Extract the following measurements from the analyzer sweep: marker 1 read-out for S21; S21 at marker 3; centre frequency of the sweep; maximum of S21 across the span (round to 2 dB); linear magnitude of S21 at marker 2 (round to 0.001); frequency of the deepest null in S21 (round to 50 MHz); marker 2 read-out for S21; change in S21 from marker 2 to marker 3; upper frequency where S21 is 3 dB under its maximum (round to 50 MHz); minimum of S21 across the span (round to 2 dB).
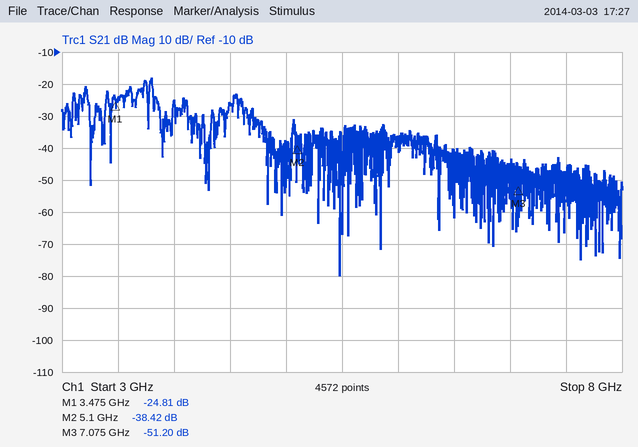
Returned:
-24.81 dB
-51.20 dB
5.5 GHz
-18 dB
0.012
5.50 GHz
-38.42 dB
-12.78 dB
3.80 GHz
-80 dB
